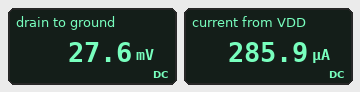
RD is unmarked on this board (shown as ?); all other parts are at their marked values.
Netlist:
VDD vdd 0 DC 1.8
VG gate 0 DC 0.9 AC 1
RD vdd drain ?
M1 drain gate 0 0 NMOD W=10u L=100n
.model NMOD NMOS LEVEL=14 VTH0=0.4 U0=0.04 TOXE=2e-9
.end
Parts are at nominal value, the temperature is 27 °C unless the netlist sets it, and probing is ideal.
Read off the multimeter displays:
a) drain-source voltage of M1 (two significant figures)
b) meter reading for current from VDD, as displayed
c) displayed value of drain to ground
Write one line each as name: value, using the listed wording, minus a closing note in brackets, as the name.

drain-source voltage of M1: 28 mV
meter reading for current from VDD, as displayed: 285.9 µA
displayed value of drain to ground: 27.6 mV
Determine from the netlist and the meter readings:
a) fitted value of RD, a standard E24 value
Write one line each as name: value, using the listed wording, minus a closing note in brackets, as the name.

fitted value of RD, a standard E24 value: 6.2 kΩ
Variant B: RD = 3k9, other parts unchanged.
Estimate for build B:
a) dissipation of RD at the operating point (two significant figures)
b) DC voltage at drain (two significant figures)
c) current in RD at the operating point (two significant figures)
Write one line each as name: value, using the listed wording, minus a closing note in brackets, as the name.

dissipation of RD at the operating point: 790 µW
DC voltage at drain: 45 mV
current in RD at the operating point: 450 µA
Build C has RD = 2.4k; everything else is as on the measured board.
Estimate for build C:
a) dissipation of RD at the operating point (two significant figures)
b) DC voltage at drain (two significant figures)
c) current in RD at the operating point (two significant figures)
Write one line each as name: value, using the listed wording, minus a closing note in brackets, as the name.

dissipation of RD at the operating point: 1.2 mW
DC voltage at drain: 77 mV
current in RD at the operating point: 720 µA
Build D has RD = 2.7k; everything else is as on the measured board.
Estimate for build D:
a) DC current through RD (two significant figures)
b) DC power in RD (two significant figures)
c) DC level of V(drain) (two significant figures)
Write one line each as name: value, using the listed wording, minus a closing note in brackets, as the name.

DC current through RD: 640 µA
DC power in RD: 1.1 mW
DC level of V(drain): 68 mV
